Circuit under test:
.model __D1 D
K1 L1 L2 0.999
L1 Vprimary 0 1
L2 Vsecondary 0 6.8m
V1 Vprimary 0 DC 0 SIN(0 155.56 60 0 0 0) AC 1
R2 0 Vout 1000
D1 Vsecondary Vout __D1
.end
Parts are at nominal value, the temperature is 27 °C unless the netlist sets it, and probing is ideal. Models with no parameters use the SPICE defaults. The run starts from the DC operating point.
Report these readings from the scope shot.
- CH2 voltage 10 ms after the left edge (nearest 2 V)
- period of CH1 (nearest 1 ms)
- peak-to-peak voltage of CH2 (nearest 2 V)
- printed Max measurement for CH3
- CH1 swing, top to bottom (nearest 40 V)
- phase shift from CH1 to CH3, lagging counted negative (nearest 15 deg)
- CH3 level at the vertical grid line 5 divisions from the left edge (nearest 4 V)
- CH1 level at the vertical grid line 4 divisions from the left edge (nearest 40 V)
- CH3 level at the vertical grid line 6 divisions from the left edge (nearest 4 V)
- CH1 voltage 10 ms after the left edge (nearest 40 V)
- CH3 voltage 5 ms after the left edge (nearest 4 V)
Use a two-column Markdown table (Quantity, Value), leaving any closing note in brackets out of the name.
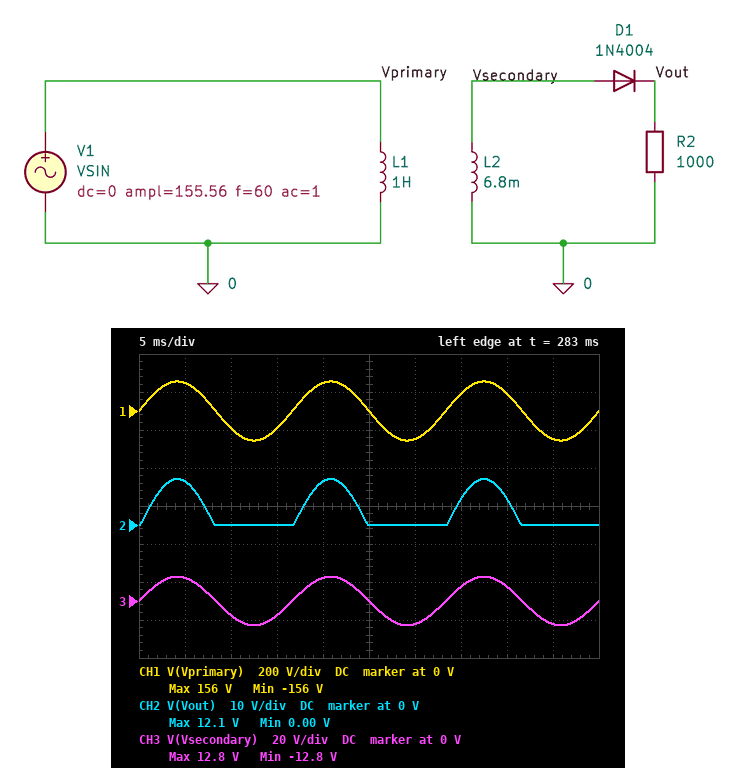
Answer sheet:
| Quantity | Value |
|---|---|
| CH2 voltage 10 ms after the left edge | 0 V |
| period of CH1 | 17 ms |
| peak-to-peak voltage of CH2 | 12 V |
| printed Max measurement for CH3 | 12.8 V |
| CH1 swing, top to bottom | 320 V |
| phase shift from CH1 to CH3, lagging counted negative | 0 deg |
| CH3 level at the vertical grid line 5 divisions from the left edge | 0 V |
| CH1 level at the vertical grid line 4 divisions from the left edge | 160 V |
| CH3 level at the vertical grid line 6 divisions from the left edge | -12 V |
| CH1 voltage 10 ms after the left edge | -80 V |
| CH3 voltage 5 ms after the left edge | 12 V |
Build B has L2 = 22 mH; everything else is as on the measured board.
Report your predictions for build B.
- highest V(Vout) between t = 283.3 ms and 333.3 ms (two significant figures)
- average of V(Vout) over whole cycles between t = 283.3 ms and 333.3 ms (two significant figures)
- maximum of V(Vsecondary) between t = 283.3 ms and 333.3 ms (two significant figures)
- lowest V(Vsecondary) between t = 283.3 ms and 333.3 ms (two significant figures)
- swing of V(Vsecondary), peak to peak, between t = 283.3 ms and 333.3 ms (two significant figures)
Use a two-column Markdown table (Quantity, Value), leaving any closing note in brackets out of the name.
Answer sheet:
| Quantity | Value |
|---|---|
| highest V(Vout) between t = 283.3 ms and 333.3 ms | 22 V |
| average of V(Vout) over whole cycles between t = 283.3 ms and 333.3 ms | 7.0 V |
| maximum of V(Vsecondary) between t = 283.3 ms and 333.3 ms | 23 V |
| lowest V(Vsecondary) between t = 283.3 ms and 333.3 ms | -23 V |
| swing of V(Vsecondary), peak to peak, between t = 283.3 ms and 333.3 ms | 46 V |
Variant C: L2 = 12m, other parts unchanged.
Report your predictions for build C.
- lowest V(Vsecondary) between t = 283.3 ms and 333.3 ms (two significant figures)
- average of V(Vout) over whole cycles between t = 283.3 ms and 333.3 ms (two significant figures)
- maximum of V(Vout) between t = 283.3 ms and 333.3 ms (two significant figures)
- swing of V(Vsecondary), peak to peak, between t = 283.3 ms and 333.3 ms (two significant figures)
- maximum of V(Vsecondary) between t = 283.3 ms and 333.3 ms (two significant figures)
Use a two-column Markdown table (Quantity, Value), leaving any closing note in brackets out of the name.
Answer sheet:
| Quantity | Value |
|---|---|
| lowest V(Vsecondary) between t = 283.3 ms and 333.3 ms | -17 V |
| average of V(Vout) over whole cycles between t = 283.3 ms and 333.3 ms | 5.1 V |
| maximum of V(Vout) between t = 283.3 ms and 333.3 ms | 16 V |
| swing of V(Vsecondary), peak to peak, between t = 283.3 ms and 333.3 ms | 34 V |
| maximum of V(Vsecondary) between t = 283.3 ms and 333.3 ms | 17 V |
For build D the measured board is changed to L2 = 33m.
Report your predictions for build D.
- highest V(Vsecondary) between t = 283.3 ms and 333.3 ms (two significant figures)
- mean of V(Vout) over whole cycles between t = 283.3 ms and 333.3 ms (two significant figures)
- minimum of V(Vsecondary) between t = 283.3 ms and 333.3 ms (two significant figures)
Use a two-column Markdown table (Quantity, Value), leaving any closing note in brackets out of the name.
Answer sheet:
| Quantity | Value |
|---|---|
| highest V(Vsecondary) between t = 283.3 ms and 333.3 ms | 28 V |
| mean of V(Vout) over whole cycles between t = 283.3 ms and 333.3 ms | 8.6 V |
| minimum of V(Vsecondary) between t = 283.3 ms and 333.3 ms | -28 V |
